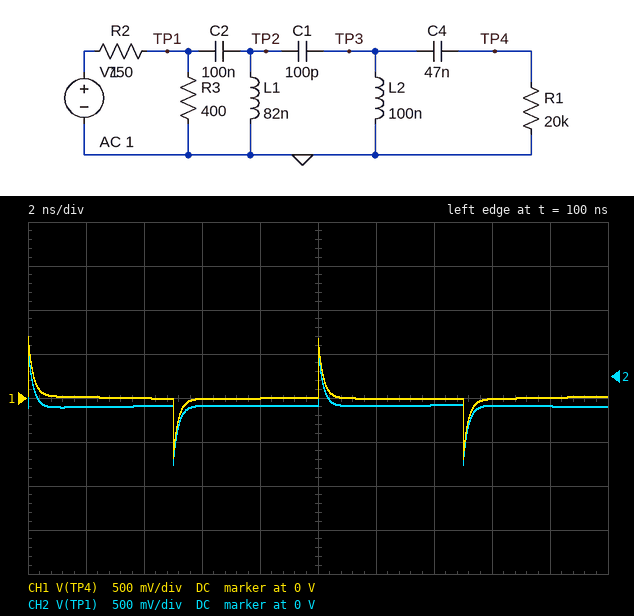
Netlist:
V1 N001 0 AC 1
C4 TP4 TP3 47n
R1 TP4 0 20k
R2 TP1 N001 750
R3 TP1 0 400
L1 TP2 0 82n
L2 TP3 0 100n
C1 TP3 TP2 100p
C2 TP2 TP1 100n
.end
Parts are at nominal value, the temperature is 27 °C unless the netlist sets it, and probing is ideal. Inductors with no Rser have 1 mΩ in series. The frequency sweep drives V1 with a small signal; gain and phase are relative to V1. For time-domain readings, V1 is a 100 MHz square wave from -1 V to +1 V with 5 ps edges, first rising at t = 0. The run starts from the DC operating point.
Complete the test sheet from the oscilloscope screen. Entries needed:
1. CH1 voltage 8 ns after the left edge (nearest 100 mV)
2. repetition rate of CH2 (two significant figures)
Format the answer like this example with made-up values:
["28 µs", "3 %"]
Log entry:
["0 V", "100 MHz"]
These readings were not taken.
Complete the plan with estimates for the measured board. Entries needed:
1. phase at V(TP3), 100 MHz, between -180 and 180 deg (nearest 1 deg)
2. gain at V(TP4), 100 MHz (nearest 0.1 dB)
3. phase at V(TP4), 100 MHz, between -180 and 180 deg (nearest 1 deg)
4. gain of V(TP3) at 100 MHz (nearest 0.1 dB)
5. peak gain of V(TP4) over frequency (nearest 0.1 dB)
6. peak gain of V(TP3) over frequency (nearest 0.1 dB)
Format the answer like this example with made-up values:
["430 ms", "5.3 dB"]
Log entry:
["85 deg", "-27.2 dB", "85 deg", "-27.2 dB", "-7.6 dB", "-7.6 dB"]
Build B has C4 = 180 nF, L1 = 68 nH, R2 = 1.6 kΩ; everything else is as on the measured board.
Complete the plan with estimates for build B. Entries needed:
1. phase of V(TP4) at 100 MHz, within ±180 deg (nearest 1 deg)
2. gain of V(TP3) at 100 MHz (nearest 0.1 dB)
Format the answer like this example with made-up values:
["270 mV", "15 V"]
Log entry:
["86 deg", "-34.6 dB"]
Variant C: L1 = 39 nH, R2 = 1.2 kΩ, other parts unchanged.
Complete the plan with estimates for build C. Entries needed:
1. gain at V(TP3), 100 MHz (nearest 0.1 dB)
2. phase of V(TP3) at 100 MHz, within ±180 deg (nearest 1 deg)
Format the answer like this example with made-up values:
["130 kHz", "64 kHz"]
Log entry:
["-34.9 dB", "87 deg"]
